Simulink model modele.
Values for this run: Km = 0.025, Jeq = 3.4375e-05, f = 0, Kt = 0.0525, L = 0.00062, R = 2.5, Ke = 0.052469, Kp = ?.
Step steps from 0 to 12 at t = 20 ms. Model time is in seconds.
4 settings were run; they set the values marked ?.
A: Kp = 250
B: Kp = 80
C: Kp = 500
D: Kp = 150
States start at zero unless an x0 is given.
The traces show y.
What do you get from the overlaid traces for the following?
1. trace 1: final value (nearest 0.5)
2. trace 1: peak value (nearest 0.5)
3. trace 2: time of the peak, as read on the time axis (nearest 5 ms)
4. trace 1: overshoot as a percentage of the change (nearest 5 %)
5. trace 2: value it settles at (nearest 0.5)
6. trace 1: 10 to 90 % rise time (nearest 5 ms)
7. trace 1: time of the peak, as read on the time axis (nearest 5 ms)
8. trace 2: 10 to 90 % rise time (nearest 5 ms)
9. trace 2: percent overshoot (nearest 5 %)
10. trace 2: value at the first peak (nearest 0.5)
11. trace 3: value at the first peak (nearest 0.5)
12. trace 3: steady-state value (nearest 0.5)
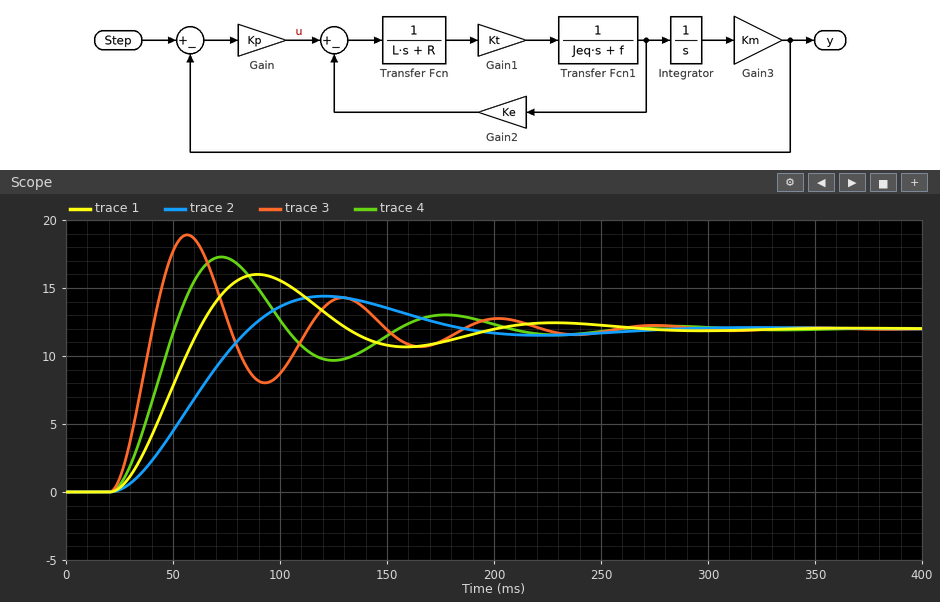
12.0
16.0
120 ms
35 %
12.0
30 ms
90 ms
45 ms
20 %
14.5
19.0
12.0
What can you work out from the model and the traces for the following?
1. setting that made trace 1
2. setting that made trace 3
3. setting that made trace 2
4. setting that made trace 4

D
C
B
A
